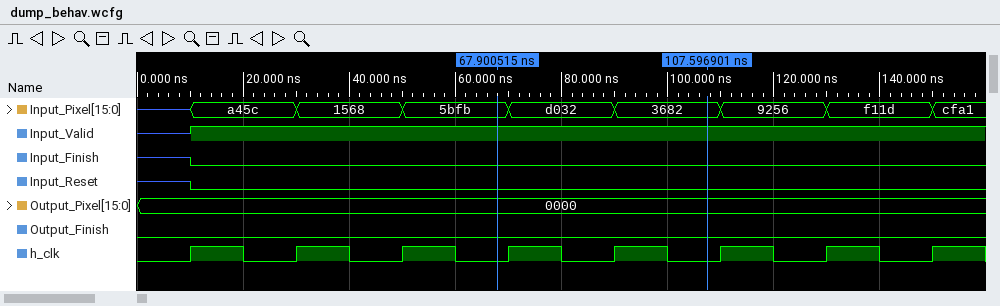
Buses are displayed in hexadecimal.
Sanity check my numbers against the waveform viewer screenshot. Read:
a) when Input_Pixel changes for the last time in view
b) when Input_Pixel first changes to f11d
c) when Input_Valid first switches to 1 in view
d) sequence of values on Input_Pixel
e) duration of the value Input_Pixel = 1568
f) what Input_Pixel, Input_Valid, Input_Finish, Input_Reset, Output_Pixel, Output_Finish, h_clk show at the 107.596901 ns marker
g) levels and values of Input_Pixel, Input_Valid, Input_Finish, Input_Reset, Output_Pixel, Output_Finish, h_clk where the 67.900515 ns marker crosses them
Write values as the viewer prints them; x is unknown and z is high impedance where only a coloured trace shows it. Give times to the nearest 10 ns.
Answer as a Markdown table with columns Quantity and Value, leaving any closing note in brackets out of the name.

| Quantity | Value |
|---|---|
| when Input_Pixel changes for the last time in view | 150 ns |
| when Input_Pixel first changes to f11d | 130 ns |
| when Input_Valid first switches to 1 in view | 10 ns |
| sequence of values on Input_Pixel | z, a45c, 1568, 5bfb, d032, 3682, 9256, f11d, cfa1 |
| duration of the value Input_Pixel = 1568 | 20 ns |
| what Input_Pixel, Input_Valid, Input_Finish, Input_Reset, Output_Pixel, Output_Finish, h_clk show at the 107.596901 ns marker | Input_Pixel=3682, Input_Valid=1, Input_Finish=0, Input_Reset=0, Output_Pixel=0000, Output_Finish=0, h_clk=0 |
| levels and values of Input_Pixel, Input_Valid, Input_Finish, Input_Reset, Output_Pixel, Output_Finish, h_clk where the 67.900515 ns marker crosses them | Input_Pixel=5bfb, Input_Valid=1, Input_Finish=0, Input_Reset=0, Output_Pixel=0000, Output_Finish=0, h_clk=0 |
